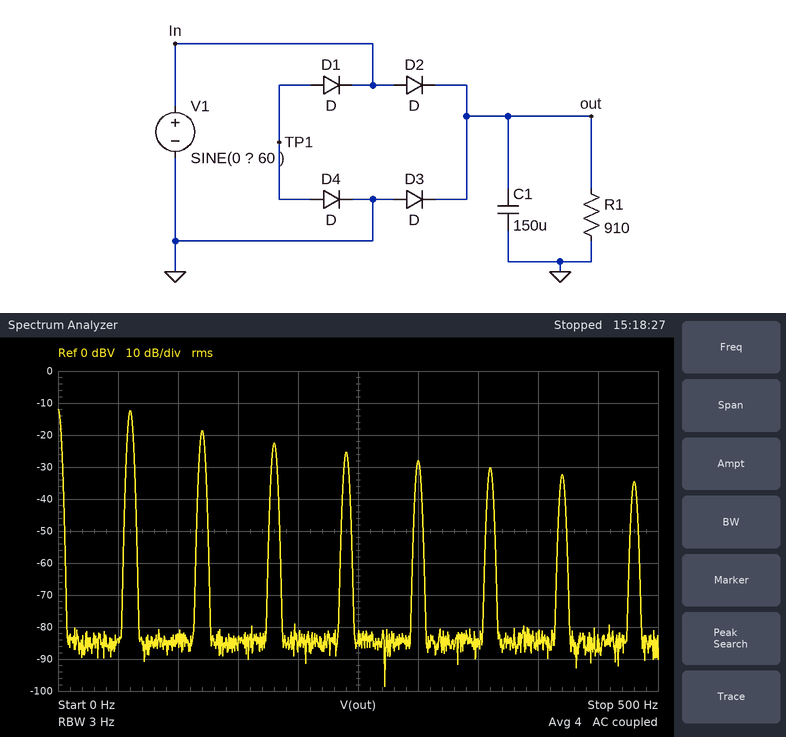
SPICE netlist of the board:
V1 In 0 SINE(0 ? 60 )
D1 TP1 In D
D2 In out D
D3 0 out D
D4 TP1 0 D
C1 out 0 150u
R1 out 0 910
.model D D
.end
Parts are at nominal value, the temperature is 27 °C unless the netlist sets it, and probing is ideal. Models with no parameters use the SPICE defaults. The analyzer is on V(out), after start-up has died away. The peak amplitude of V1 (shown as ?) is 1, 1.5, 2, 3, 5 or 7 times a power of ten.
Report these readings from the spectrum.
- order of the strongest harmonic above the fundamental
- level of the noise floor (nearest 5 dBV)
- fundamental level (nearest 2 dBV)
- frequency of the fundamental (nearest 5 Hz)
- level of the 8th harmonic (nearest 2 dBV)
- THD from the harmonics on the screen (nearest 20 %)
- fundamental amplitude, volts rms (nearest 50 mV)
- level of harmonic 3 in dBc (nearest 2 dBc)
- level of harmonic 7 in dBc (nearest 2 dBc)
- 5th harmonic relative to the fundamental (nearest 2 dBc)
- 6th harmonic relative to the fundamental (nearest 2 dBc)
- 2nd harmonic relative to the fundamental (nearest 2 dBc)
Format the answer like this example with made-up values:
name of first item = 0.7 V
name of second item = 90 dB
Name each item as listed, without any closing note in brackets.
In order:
order of the strongest harmonic above the fundamental = 2
level of the noise floor = -85 dBV
fundamental level = -12 dBV
frequency of the fundamental = 60 Hz
level of the 8th harmonic = -34 dBV
THD from the harmonics on the screen = 60 %
fundamental amplitude, volts rms = 250 mV
level of harmonic 3 in dBc = -10 dBc
level of harmonic 7 in dBc = -20 dBc
5th harmonic relative to the fundamental = -16 dBc
6th harmonic relative to the fundamental = -18 dBc
2nd harmonic relative to the fundamental = -6 dBc
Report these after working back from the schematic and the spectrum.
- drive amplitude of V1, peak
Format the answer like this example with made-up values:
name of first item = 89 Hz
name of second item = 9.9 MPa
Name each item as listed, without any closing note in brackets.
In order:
drive amplitude of V1, peak = 10 V
